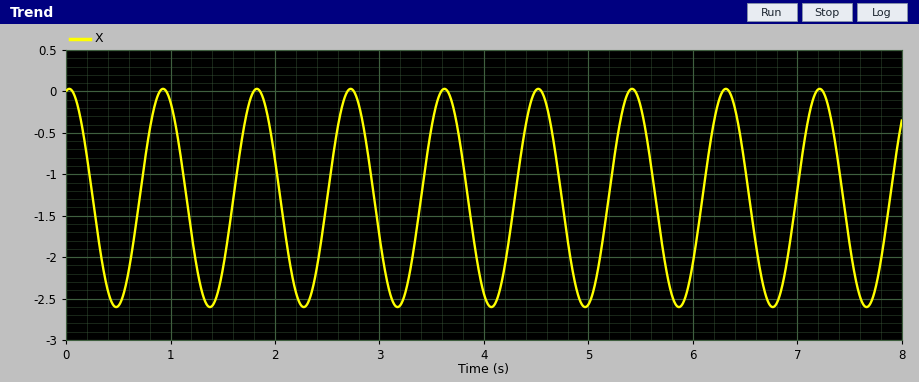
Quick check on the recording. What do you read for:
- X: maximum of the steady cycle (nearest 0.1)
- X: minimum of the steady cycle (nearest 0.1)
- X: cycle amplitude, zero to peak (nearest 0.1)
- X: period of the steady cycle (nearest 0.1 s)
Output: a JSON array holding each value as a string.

["0.0", "-2.6", "1.3", "0.9 s"]
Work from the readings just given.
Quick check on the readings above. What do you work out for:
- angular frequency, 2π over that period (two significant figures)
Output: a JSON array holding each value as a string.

["7.0 rad/s"]
